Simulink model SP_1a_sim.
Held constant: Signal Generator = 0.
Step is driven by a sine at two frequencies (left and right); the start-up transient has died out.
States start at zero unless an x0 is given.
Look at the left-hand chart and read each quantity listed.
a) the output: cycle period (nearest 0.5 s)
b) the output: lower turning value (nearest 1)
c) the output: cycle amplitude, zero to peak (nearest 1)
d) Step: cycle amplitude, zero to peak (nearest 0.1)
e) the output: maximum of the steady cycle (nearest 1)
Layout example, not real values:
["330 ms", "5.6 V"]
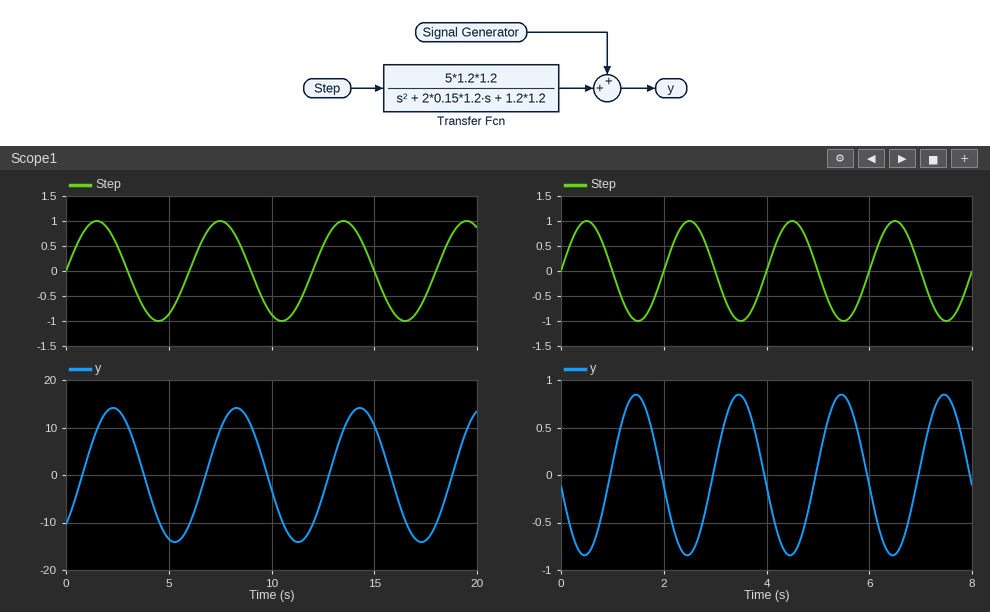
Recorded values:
["6.0 s", "-14", "14", "1.0", "14"]
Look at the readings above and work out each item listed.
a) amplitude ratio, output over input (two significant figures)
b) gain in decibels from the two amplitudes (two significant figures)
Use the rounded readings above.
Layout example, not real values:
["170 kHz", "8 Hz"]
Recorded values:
["14", "23 dB"]
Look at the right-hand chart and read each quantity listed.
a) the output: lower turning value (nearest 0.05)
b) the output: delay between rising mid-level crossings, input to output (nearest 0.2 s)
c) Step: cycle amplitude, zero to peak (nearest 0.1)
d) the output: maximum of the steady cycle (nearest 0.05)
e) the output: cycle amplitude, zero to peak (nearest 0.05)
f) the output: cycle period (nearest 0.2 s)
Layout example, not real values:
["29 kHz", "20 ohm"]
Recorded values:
["-0.85", "1.0 s", "1.0", "0.85", "0.85", "2.0 s"]
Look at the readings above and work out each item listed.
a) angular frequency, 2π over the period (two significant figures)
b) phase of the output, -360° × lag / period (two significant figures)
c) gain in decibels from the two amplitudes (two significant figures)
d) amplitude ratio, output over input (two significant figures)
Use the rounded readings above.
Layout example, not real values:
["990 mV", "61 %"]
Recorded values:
["3.1 rad/s", "-180°", "-1.4 dB", "0.85"]
